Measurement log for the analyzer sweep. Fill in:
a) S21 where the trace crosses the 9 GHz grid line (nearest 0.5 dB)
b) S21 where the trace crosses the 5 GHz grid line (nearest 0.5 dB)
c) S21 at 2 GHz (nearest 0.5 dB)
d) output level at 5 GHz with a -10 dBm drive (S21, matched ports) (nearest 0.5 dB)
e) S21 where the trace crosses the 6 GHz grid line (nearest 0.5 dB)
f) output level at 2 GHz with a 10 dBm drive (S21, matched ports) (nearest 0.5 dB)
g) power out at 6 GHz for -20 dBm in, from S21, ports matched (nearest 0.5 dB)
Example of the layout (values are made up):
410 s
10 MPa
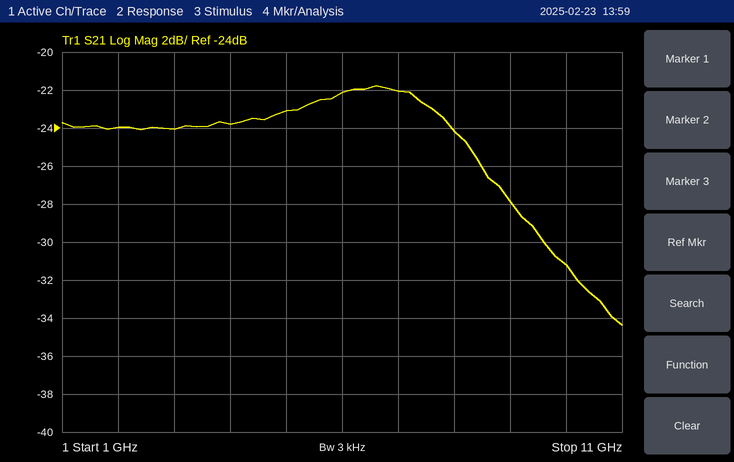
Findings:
-28.0 dB
-23.0 dB
-24.0 dB
-33.0 dBm
-22.0 dB
-14.0 dBm
-42.0 dBm
